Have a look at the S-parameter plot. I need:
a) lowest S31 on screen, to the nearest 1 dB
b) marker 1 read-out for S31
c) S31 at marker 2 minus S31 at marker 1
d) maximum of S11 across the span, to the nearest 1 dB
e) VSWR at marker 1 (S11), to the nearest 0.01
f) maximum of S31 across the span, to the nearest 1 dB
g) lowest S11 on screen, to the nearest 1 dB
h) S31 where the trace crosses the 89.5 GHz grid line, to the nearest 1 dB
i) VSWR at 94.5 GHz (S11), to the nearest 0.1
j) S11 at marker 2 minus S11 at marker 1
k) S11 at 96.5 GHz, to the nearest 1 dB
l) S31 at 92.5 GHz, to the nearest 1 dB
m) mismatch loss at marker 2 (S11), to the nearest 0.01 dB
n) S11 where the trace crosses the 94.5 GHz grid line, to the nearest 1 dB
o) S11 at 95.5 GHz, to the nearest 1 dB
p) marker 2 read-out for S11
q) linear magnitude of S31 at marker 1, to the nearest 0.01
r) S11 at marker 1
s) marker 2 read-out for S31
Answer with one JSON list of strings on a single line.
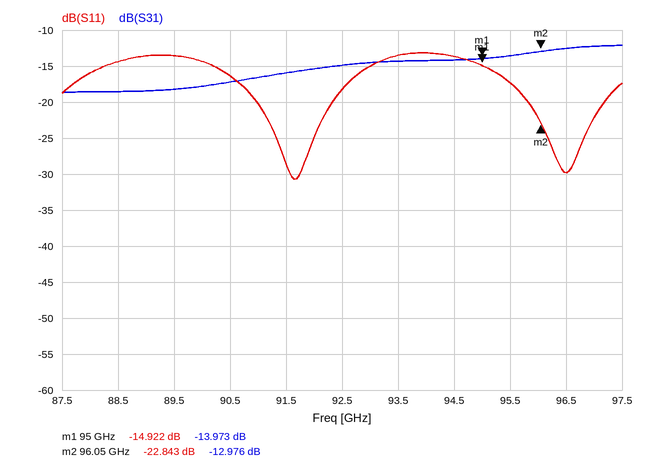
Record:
["-19 dB", "-13.973 dB", "0.997 dB", "-13 dB", "1.44", "-12 dB", "-31 dB", "-18 dB", "1.5", "-7.921 dB", "-30 dB", "-15 dB", "0.02 dB", "-14 dB", "-17 dB", "-22.843 dB", "0.20", "-14.922 dB", "-12.976 dB"]
